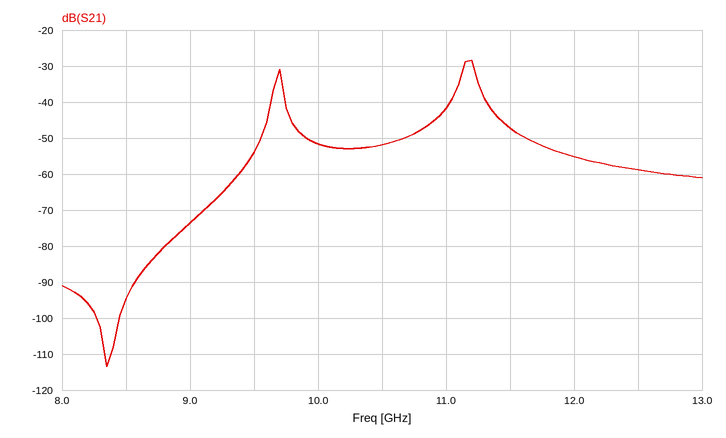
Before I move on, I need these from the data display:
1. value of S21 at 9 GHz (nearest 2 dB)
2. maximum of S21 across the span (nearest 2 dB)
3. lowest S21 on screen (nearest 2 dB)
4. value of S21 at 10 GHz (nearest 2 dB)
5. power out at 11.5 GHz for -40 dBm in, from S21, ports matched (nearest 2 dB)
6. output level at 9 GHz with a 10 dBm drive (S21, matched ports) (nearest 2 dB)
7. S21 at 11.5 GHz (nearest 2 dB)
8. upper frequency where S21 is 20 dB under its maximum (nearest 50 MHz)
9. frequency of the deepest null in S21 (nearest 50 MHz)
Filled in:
-74 dB
-28 dB
-114 dB
-52 dB
-88 dBm
-64 dBm
-48 dB
11.55 GHz
8.35 GHz
